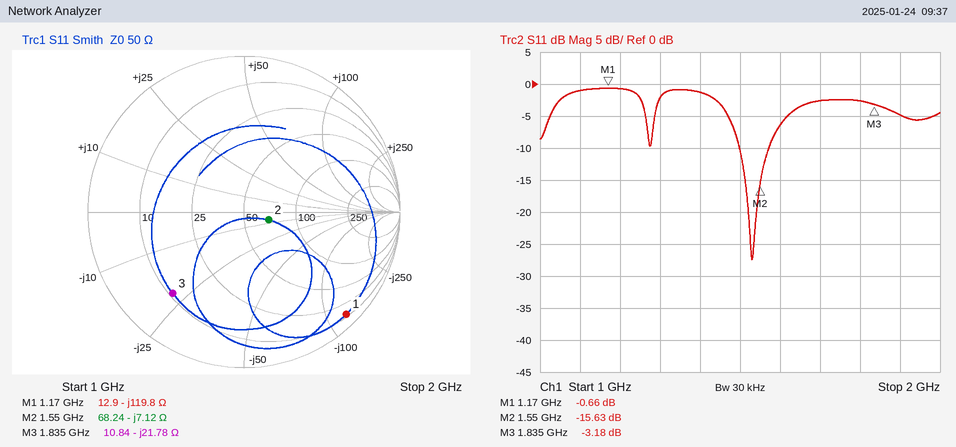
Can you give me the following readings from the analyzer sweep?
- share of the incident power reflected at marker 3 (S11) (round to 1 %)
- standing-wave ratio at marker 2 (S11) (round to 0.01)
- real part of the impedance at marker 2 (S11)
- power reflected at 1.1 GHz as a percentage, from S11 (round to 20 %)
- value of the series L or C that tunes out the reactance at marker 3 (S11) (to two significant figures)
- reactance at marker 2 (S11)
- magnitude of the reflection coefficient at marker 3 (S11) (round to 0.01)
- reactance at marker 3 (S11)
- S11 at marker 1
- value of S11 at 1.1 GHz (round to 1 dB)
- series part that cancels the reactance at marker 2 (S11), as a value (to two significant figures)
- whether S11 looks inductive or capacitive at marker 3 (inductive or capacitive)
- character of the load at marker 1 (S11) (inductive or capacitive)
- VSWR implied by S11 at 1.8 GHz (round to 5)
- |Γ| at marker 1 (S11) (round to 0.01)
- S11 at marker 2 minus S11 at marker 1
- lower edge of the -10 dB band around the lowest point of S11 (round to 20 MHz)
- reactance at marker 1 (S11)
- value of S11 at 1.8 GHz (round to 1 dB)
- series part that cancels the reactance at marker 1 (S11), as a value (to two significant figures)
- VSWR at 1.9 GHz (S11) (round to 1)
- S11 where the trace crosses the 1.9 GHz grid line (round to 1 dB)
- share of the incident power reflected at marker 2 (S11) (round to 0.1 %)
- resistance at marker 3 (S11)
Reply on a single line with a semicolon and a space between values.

48 %; 1.40; 68.24 Ω; 80 %; 1.9 nH; -7.12 Ω; 0.69; -21.78 Ω; -0.66 dB; -1 dB; 730 pH; capacitive; capacitive; 5; 0.93; -14.97 dB; 1.50 GHz; -119.8 Ω; -3 dB; 16 nH; 4; -5 dB; 2.7 %; 10.84 Ω
